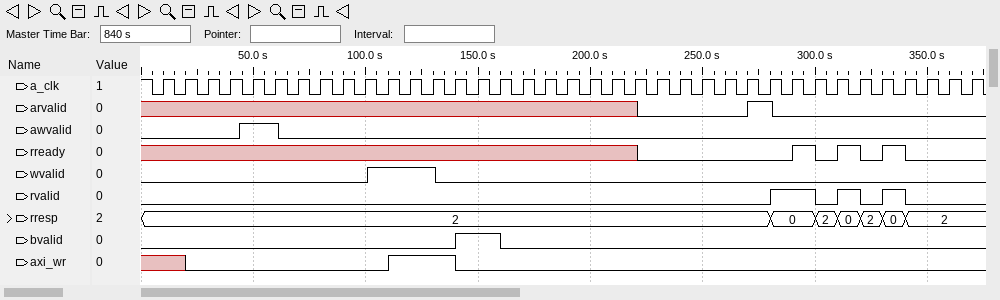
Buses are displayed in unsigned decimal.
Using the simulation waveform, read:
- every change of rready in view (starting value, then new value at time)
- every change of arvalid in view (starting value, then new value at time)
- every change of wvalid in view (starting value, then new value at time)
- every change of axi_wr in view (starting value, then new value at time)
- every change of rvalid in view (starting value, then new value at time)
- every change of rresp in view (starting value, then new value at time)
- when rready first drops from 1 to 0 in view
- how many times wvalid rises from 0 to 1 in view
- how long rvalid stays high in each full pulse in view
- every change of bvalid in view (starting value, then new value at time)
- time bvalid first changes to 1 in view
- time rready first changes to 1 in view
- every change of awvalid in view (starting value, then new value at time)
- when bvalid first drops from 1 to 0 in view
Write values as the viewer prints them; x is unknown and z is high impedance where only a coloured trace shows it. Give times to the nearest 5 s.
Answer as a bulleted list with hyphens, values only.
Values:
- x, 0 at 220 s, 1 at 290 s, 0 at 300 s, 1 at 310 s, 0 at 320 s, 1 at 330 s, 0 at 340 s
- x, 0 at 220 s, 1 at 270 s, 0 at 280 s
- 0, 1 at 100 s, 0 at 130 s
- x, 0 at 20 s, 1 at 110 s, 0 at 140 s
- 0, 1 at 280 s, 0 at 300 s, 1 at 310 s, 0 at 320 s, 1 at 330 s, 0 at 340 s
- 2, 0 at 280 s, 2 at 300 s, 0 at 310 s, 2 at 320 s, 0 at 330 s, 2 at 340 s
- 300 s
- 1
- 20 s, 10 s, 10 s
- 0, 1 at 140 s, 0 at 160 s
- 140 s
- 290 s
- 0, 1 at 45 s, 0 at 60 s
- 160 s
